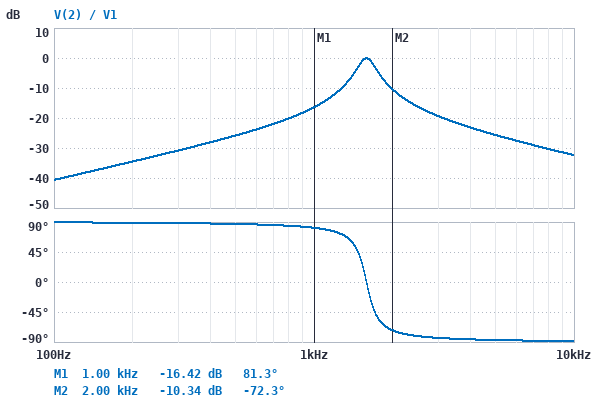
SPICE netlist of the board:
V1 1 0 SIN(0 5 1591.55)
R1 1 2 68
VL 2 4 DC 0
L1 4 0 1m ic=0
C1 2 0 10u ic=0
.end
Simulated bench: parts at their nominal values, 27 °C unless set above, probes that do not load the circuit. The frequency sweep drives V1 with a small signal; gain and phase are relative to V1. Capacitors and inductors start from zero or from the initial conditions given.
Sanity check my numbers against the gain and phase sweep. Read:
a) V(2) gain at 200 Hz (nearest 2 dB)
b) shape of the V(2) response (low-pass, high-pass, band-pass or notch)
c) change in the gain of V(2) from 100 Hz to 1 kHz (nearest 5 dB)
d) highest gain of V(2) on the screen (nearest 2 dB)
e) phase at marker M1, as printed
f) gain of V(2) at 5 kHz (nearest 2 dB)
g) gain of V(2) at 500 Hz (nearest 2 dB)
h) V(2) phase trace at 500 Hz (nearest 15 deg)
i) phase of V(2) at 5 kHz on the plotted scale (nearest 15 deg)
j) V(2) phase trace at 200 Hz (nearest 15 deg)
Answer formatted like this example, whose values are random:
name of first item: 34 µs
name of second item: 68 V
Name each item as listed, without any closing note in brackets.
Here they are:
V(2) gain at 200 Hz: -34 dB
shape of the V(2) response: band-pass
change in the gain of V(2) from 100 Hz to 1 kHz: 25 dB
highest gain of V(2) on the screen: 0 dB
phase at marker M1, as printed: 81.3 deg
gain of V(2) at 5 kHz: -26 dB
gain of V(2) at 500 Hz: -26 dB
V(2) phase trace at 500 Hz: 90 deg
phase of V(2) at 5 kHz on the plotted scale: -90 deg
V(2) phase trace at 200 Hz: 90 deg
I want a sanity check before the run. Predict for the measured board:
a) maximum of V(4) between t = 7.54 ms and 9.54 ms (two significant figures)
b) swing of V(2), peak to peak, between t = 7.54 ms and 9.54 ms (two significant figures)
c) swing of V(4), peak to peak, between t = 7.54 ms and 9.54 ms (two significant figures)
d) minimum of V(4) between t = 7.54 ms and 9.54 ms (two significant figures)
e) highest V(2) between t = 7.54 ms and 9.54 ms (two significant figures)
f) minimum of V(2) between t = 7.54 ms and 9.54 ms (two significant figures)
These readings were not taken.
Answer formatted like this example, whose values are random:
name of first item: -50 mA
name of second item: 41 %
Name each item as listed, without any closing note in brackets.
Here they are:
maximum of V(4) between t = 7.54 ms and 9.54 ms: 5.0 V
swing of V(2), peak to peak, between t = 7.54 ms and 9.54 ms: 10 V
swing of V(4), peak to peak, between t = 7.54 ms and 9.54 ms: 10 V
minimum of V(4) between t = 7.54 ms and 9.54 ms: -5.0 V
highest V(2) between t = 7.54 ms and 9.54 ms: 5.0 V
minimum of V(2) between t = 7.54 ms and 9.54 ms: -5.0 V
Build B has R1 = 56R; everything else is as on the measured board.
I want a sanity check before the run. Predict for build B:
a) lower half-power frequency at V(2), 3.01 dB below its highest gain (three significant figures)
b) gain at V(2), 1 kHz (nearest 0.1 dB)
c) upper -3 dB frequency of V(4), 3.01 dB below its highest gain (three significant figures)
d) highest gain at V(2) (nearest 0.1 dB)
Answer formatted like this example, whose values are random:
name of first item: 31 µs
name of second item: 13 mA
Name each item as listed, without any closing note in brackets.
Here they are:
lower half-power frequency at V(2), 3.01 dB below its highest gain: 1.46 kHz
gain at V(2), 1 kHz: -14.8 dB
upper -3 dB frequency of V(4), 3.01 dB below its highest gain: 1.74 kHz
highest gain at V(2): 0 dB
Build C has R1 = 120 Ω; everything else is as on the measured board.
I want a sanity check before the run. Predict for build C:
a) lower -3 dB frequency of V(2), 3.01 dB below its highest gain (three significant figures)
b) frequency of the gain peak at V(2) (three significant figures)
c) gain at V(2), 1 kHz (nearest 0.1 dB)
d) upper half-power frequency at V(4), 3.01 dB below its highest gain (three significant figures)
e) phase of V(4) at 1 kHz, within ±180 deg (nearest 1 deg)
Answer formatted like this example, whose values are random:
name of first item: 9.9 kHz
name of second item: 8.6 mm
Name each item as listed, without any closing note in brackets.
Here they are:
lower -3 dB frequency of V(2), 3.01 dB below its highest gain: 1.53 kHz
frequency of the gain peak at V(2): 1.59 kHz
gain at V(2), 1 kHz: -21.3 dB
upper half-power frequency at V(4), 3.01 dB below its highest gain: 1.66 kHz
phase of V(4) at 1 kHz, within ±180 deg: 85 deg
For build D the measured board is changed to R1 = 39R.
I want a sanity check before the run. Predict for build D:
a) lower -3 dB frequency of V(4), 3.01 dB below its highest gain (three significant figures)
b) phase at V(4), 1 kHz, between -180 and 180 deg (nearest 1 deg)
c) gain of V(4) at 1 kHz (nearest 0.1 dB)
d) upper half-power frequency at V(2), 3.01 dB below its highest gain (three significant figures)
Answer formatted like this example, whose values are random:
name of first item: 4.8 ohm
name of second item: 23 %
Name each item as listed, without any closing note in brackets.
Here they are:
lower -3 dB frequency of V(4), 3.01 dB below its highest gain: 1.40 kHz
phase at V(4), 1 kHz, between -180 and 180 deg: 75 deg
gain of V(4) at 1 kHz: -11.8 dB
upper half-power frequency at V(2), 3.01 dB below its highest gain: 1.81 kHz
